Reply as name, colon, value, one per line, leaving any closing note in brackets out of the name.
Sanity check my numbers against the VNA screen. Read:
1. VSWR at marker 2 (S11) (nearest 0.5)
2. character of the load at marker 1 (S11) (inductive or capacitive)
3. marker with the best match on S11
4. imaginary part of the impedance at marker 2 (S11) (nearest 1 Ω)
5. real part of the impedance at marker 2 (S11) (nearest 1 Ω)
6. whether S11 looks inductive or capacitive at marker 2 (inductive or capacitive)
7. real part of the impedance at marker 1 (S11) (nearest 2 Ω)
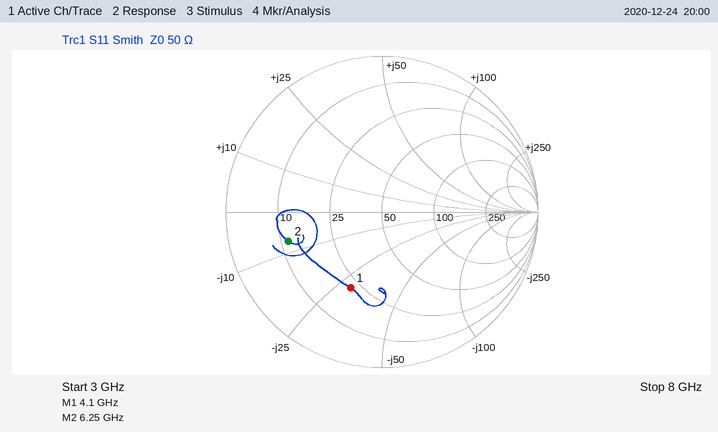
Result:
VSWR at marker 2 (S11): 4.5
character of the load at marker 1 (S11): capacitive
marker with the best match on S11: marker 1
imaginary part of the impedance at marker 2 (S11): -7 Ω
real part of the impedance at marker 2 (S11): 12 Ω
whether S11 looks inductive or capacitive at marker 2: capacitive
real part of the impedance at marker 1 (S11): 22 Ω
